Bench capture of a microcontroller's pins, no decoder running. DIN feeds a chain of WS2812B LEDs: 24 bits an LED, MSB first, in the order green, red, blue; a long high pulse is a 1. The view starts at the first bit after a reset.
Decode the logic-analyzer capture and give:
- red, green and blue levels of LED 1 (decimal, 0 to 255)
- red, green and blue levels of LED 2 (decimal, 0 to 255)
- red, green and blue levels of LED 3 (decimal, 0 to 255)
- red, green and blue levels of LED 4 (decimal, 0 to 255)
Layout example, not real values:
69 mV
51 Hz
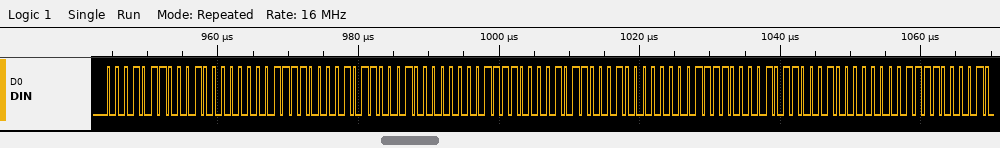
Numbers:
32, 22, 30
32, 22, 30
32, 22, 30
32, 22, 30
